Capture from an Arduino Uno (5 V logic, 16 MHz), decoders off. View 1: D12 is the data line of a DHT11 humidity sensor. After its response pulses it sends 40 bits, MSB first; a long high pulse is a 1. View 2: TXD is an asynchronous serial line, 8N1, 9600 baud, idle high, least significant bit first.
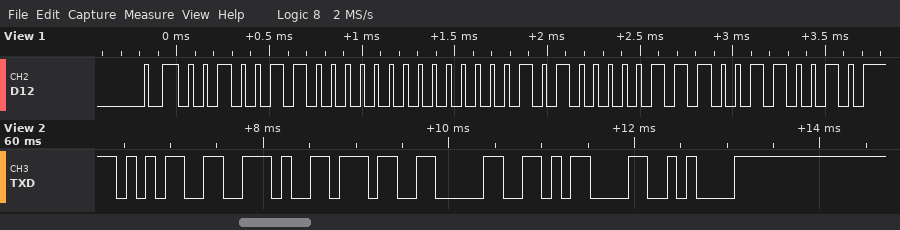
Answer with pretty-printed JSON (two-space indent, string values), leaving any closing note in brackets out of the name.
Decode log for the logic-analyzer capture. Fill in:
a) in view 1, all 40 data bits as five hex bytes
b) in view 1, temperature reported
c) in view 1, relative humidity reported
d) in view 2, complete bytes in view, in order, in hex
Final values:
{
  "in view 1, all 40 data bits as five hex bytes": "26 00 05 07 32",
  "in view 1, temperature reported": "5.7 °C",
  "in view 1, relative humidity reported": "38 %",
  "in view 2, complete bytes in view, in order, in hex": "35 2E 37 30 0D 0A"
}
